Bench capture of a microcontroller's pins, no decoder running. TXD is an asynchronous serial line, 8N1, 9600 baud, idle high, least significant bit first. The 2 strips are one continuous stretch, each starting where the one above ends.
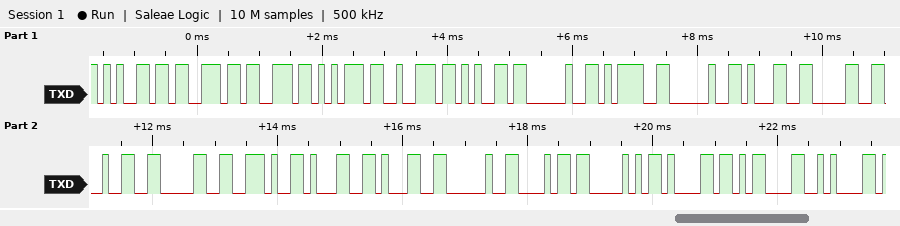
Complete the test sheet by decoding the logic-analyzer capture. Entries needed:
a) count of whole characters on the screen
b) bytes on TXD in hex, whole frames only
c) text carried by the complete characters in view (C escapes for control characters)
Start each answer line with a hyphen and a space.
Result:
- 22
- 65 73 73 75 72 65 20 3D 20 31 30 32 30 2E 31 31 20 68 50 61 0D 0A
- "essure = 1020.11 hPa\r\n"
